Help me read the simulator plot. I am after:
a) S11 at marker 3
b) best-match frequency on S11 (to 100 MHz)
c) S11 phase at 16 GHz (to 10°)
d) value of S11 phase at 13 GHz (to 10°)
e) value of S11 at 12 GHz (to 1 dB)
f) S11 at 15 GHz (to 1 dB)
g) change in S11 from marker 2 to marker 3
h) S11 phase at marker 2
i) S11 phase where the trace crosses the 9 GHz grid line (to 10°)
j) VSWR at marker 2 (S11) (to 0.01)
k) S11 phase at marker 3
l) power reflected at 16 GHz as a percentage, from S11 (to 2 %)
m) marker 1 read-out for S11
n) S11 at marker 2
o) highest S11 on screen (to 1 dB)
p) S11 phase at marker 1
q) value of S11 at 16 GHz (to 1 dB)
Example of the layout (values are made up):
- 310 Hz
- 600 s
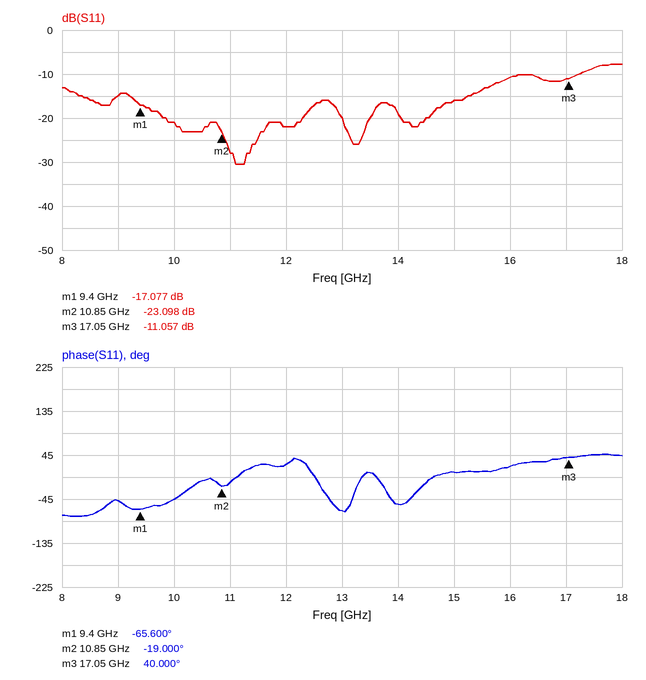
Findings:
- -11.057 dB
- 11.1 GHz
- 20°
- -70°
- -22 dB
- -16 dB
- 12.041 dB
- -19.000°
- -50°
- 1.15
- 40.000°
- 8 %
- -17.077 dB
- -23.098 dB
- -8 dB
- -65.600°
- -11 dB
